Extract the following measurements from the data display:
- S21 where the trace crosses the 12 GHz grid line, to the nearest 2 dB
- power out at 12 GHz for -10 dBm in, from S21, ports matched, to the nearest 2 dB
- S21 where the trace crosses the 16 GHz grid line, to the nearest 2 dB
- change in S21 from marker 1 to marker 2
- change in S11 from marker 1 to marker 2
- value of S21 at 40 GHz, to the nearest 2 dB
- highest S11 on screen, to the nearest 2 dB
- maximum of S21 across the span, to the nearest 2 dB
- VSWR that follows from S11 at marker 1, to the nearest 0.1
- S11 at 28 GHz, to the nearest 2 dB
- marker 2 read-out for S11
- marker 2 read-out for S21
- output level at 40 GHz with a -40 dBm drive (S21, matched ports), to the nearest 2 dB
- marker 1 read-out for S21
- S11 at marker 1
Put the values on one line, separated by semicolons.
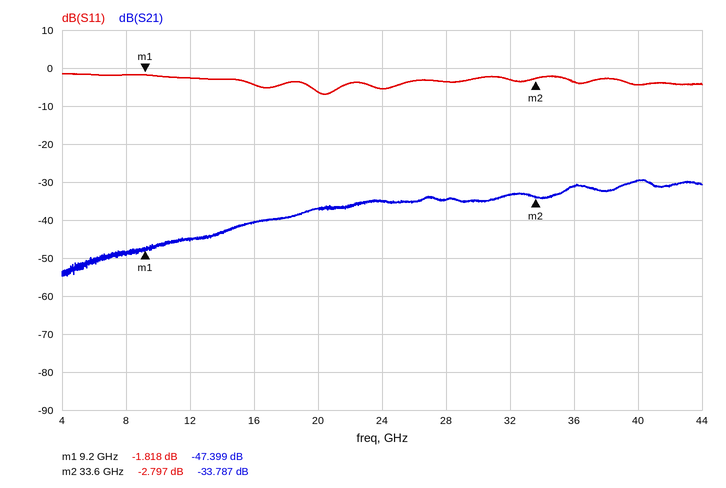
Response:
-46 dB; -56 dBm; -40 dB; 13.612 dB; -0.979 dB; -30 dB; -2 dB; -30 dB; 9.6; -4 dB; -2.797 dB; -33.787 dB; -70 dBm; -47.399 dB; -1.818 dB
